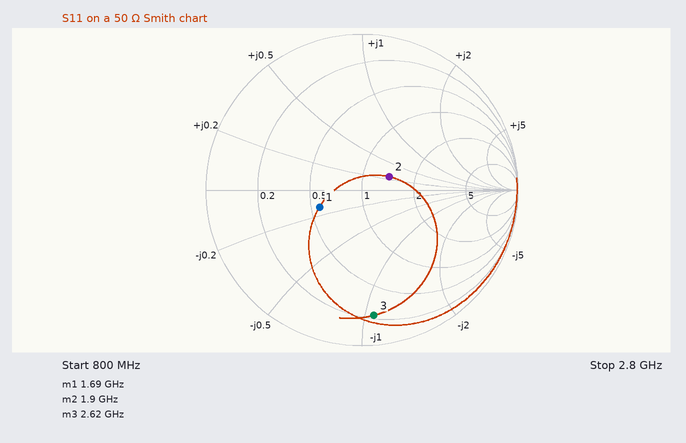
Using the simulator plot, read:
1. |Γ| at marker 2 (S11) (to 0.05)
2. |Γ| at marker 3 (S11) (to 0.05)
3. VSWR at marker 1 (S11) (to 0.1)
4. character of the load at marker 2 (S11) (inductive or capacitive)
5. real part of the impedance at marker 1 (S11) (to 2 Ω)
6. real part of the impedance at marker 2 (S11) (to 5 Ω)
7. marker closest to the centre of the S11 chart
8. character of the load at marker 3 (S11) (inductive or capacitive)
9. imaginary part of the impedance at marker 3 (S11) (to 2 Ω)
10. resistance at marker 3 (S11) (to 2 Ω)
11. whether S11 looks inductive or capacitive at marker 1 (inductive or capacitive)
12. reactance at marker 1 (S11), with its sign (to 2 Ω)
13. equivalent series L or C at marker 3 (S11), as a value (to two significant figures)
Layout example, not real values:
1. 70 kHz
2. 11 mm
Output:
1. 0.20
2. 0.80
3. 1.8
4. inductive
5. 28 Ω
6. 70 Ω
7. marker 2
8. capacitive
9. -54 Ω
10. 12 Ω
11. capacitive
12. -6 Ω
13. 1.1 pF
